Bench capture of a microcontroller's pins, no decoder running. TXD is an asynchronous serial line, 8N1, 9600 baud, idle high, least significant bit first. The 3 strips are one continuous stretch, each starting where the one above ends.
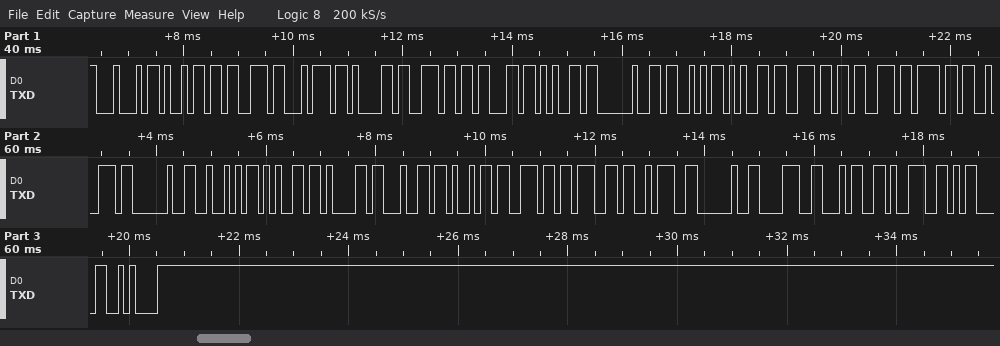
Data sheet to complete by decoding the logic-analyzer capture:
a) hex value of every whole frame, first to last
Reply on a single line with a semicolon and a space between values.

44 69 73 74 61 6E 63 65 20 53 65 6E 73 6F 72 20 52 65 61 64 69 6E 67 3A 20 38 34 39 0D 0A
